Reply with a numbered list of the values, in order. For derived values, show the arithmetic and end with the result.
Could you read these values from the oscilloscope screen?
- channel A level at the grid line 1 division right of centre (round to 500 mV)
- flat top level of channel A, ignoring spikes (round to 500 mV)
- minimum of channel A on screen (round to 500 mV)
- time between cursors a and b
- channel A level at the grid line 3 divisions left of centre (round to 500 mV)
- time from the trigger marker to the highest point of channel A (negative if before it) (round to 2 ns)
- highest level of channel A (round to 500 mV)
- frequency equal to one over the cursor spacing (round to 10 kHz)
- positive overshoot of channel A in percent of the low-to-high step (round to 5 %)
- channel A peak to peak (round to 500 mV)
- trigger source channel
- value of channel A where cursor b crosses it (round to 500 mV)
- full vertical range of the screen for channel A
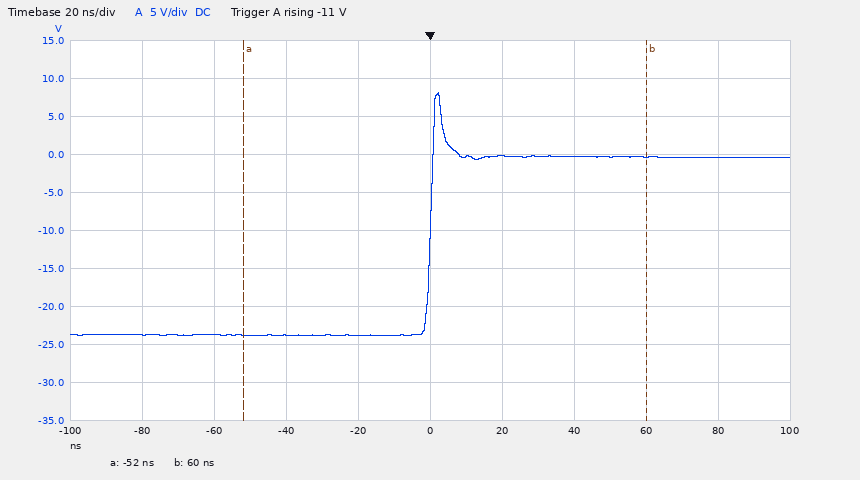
1. 0.0 V
2. -500 mV
3. -24.0 V
4. 60 ns − (-52 ns) = 112 ns
5. -23.5 V
6. +2 ns
7. 8.0 V
8. 1 / 112 ns ≈ 8.93 MHz
9. 35 %
10. 8.0 V − (-24.0 V) = 32.0 V
11. channel A
12. -500 mV
13. 50 V
